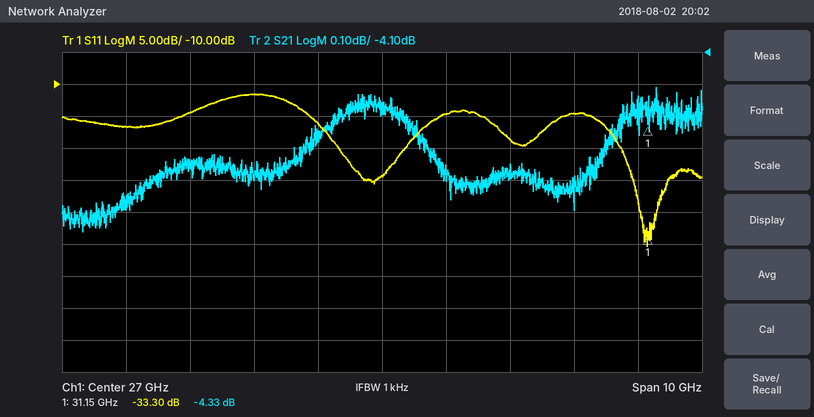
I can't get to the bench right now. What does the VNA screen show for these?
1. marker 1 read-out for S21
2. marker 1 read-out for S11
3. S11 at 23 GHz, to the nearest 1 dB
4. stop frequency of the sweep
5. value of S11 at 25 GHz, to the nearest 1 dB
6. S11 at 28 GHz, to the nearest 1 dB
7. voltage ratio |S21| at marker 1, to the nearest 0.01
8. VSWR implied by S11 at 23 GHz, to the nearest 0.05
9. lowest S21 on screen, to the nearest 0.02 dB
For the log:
-4.33 dB
-33.30 dB
-17 dB
32 GHz
-12 dB
-15 dB
0.61
1.35
-4.66 dB
